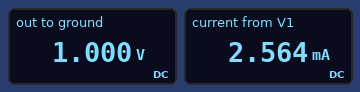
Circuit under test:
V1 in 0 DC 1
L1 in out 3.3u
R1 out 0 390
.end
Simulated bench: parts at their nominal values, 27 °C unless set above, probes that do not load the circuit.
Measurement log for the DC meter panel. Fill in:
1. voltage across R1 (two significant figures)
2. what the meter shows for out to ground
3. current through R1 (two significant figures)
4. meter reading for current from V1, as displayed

1.0 V
1.000 V
2.6 mA
2.564 mA
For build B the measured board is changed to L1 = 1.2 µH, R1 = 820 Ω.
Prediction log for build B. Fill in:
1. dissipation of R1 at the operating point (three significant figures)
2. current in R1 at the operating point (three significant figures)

1.22 mW
1.22 mA
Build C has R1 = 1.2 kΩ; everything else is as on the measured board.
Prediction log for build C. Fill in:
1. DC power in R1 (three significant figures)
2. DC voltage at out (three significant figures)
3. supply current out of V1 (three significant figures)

833 µW
1.00 V
833 µA
